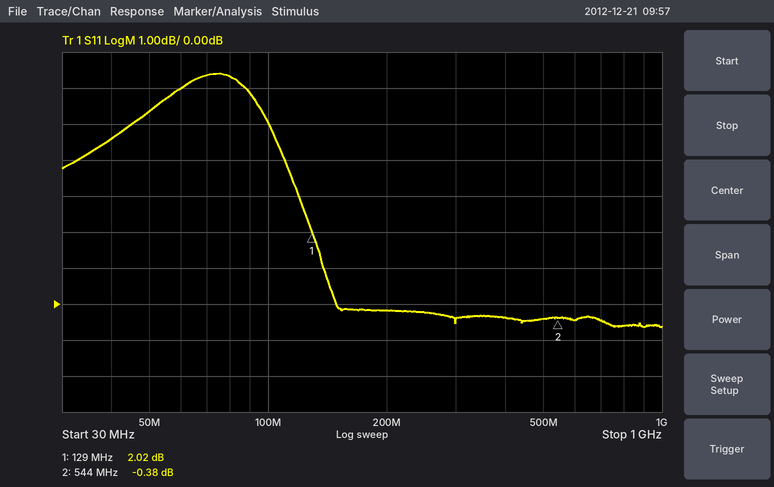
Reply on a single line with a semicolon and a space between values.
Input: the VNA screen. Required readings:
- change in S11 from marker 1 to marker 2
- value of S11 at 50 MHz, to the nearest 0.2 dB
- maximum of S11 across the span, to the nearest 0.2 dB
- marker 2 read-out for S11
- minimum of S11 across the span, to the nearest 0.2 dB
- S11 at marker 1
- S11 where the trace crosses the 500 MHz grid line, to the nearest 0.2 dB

-2.40 dB; 5.4 dB; 6.4 dB; -0.38 dB; -0.6 dB; 2.02 dB; -0.4 dB
